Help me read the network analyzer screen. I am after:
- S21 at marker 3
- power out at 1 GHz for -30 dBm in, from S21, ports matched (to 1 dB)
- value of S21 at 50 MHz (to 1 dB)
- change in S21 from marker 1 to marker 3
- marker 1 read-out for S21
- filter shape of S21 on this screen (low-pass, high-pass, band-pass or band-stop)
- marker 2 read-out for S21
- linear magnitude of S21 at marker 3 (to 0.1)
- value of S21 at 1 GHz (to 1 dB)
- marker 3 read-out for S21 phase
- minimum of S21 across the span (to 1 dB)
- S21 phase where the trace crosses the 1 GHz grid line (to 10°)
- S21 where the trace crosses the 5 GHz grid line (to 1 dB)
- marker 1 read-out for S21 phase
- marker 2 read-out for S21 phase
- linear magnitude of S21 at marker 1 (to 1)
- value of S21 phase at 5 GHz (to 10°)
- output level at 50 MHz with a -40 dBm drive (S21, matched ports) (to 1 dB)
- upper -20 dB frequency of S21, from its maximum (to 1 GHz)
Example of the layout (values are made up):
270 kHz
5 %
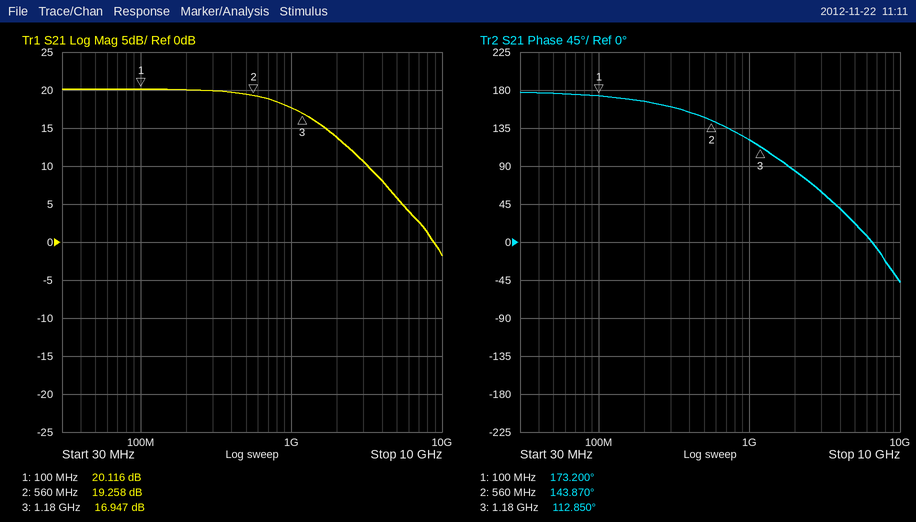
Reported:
16.947 dB
-12 dBm
20 dB
-3.169 dB
20.116 dB
low-pass
19.258 dB
7.0
18 dB
112.850°
-2 dB
120°
6 dB
173.200°
143.870°
10
20°
-20 dBm
9 GHz
